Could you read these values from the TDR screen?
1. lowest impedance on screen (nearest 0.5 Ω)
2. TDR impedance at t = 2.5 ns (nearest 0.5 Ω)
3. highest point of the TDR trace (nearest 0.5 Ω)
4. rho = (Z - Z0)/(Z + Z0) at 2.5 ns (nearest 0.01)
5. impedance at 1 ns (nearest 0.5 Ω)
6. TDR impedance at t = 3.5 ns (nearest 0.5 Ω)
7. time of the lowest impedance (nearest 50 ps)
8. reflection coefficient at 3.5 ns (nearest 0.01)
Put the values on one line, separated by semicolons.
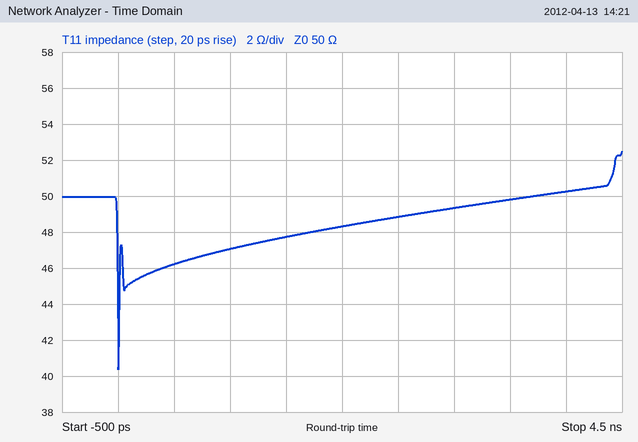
40.5 Ω; 49.0 Ω; 52.5 Ω; -0.01; 47.0 Ω; 50.0 Ω; 0 ps; 0.00
